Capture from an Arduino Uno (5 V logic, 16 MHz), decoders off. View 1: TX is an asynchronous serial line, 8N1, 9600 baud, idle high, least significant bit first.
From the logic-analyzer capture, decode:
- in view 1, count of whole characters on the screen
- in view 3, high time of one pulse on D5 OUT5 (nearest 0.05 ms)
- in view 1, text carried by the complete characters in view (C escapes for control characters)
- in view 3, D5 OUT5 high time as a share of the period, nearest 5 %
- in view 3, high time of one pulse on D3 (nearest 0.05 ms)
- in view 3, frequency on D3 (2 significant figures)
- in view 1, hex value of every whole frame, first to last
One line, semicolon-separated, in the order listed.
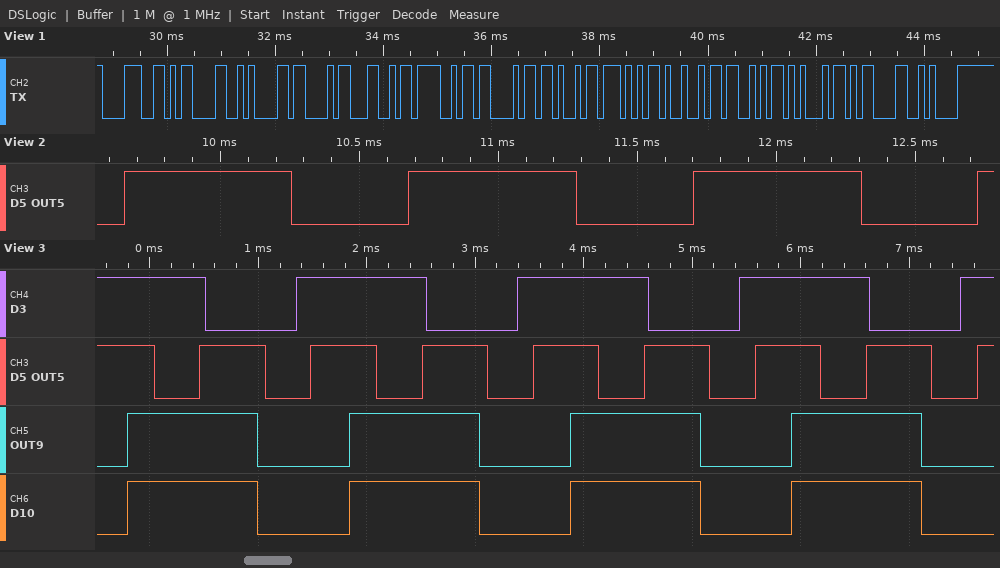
14; 0.60 ms; "8\r\nCLOCKWISE\r\n"; 60 %; 1.20 ms; 490 Hz; 0x38 0x0D 0x0A 0x43 0x4C 0x4F 0x43 0x4B 0x57 0x49 0x53 0x45 0x0D 0x0A
